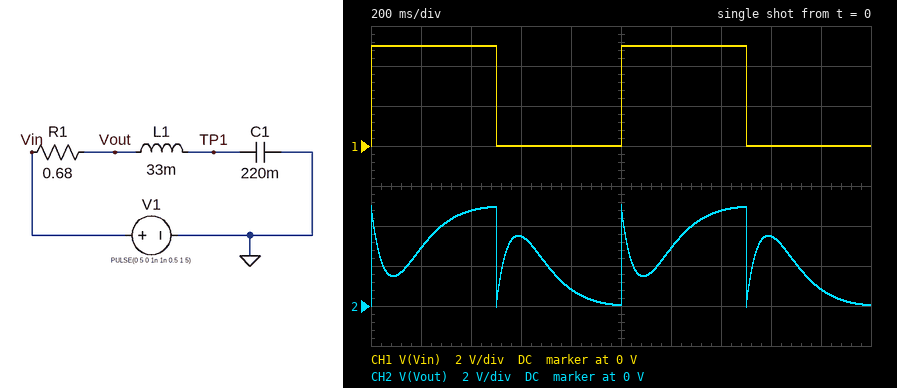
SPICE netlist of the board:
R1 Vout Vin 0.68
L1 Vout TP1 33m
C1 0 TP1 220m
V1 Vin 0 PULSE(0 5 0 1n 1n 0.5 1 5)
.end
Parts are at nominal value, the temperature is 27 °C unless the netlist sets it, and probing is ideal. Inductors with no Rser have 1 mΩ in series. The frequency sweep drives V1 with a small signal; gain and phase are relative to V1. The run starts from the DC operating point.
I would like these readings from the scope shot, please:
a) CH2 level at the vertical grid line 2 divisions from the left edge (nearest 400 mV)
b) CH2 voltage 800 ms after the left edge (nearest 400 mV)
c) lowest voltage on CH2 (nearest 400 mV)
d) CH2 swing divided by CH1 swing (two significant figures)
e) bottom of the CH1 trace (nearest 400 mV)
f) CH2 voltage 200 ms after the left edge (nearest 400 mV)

4.8 V
800 mV
0 V
1.0
0 V
2.8 V
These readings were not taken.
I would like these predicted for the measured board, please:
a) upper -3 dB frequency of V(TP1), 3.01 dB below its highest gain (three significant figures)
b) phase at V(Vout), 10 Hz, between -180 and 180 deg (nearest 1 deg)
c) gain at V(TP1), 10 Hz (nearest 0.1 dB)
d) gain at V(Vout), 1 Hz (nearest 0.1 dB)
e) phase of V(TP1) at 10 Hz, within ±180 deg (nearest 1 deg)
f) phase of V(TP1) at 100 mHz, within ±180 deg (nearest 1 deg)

1.44 Hz
19 deg
-29.3 dB
-4.4 dB
-161 deg
-5 deg
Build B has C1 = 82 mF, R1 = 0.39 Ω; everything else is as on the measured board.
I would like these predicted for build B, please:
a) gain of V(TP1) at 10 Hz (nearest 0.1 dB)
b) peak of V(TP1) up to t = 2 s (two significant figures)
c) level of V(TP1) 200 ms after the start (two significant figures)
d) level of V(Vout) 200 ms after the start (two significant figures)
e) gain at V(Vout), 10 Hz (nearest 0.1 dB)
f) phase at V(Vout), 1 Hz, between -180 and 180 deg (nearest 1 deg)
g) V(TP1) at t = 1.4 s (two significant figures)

-19.9 dB
6.9 V
6.6 V
5.5 V
-0.2 dB
-13 deg
4.6 V
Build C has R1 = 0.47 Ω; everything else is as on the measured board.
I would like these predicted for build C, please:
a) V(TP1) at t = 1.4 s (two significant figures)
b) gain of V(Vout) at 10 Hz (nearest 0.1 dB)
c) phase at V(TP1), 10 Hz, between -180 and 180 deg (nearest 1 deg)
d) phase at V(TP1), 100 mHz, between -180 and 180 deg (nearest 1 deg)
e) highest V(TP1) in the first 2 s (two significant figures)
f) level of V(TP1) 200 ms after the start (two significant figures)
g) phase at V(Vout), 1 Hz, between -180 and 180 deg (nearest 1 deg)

5.4 V
-0.2 dB
-167 deg
-4 deg
5.5 V
4.5 V
-42 deg
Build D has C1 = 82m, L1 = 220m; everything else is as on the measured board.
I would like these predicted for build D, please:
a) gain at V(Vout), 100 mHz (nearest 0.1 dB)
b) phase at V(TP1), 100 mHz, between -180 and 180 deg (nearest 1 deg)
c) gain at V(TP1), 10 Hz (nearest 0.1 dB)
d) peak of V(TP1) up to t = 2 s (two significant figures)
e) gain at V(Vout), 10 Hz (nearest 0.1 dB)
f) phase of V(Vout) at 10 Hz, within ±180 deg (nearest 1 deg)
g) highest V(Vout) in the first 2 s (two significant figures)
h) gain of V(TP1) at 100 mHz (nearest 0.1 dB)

0 dB
-2 deg
-36.9 dB
9.3 V
0 dB
3 deg
6.1 V
0.1 dB
